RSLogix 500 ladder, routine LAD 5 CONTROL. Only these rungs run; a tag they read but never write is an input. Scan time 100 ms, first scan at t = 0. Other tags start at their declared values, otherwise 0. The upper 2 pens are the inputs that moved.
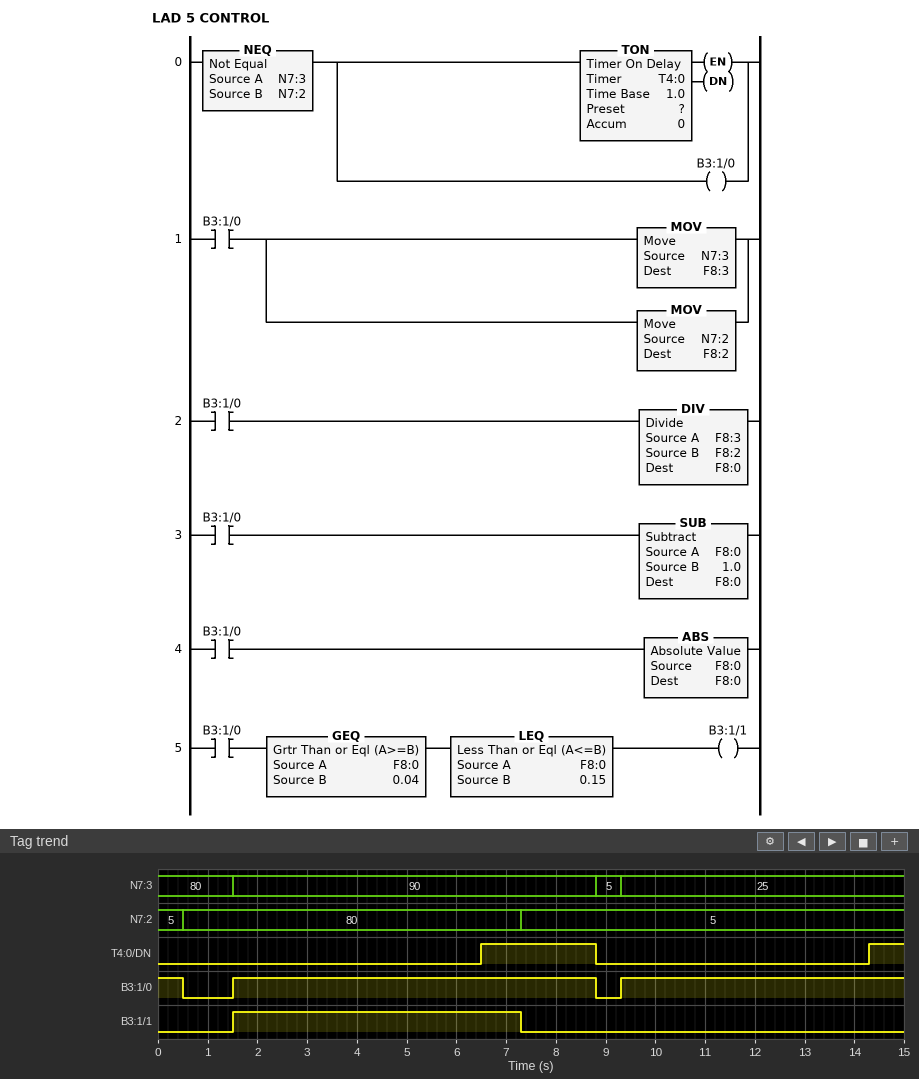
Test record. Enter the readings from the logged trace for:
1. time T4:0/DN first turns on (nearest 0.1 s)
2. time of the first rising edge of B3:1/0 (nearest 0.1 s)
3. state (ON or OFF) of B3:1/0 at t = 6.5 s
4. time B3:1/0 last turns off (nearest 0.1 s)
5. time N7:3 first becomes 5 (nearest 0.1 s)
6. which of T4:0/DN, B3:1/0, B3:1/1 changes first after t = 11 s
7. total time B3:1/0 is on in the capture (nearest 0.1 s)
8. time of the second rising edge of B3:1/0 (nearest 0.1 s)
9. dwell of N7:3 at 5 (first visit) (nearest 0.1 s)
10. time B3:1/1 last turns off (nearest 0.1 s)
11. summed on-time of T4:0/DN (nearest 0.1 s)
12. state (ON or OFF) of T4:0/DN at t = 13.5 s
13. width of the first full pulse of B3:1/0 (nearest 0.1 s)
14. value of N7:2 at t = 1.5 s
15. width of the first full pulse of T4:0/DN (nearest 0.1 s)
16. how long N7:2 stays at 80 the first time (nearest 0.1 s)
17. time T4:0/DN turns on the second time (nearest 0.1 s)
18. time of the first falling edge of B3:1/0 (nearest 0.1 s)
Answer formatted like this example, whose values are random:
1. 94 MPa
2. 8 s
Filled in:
1. 6.5 s
2. 1.5 s
3. ON
4. 8.8 s
5. 8.8 s
6. T4:0/DN
7. 13.5 s
8. 9.3 s
9. 0.5 s
10. 7.3 s
11. 3.0 s
12. OFF
13. 7.3 s
14. 80
15. 2.3 s
16. 6.8 s
17. 14.3 s
18. 0.5 s
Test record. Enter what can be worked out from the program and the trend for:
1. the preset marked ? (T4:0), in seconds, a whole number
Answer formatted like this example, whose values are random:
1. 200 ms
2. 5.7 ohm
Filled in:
1. 5 s
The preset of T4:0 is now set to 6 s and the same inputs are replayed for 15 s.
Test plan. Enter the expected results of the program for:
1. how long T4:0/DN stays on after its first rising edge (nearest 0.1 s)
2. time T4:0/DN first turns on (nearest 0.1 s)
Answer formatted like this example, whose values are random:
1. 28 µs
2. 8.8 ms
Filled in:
1. 1.3 s
2. 7.5 s
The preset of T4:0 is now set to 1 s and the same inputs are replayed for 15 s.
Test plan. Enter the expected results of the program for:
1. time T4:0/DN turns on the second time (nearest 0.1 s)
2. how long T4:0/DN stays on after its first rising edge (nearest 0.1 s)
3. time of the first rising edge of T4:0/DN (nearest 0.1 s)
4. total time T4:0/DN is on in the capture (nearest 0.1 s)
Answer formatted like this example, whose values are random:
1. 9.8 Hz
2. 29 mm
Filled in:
1. 10.3 s
2. 6.3 s
3. 2.5 s
4. 11.0 s
